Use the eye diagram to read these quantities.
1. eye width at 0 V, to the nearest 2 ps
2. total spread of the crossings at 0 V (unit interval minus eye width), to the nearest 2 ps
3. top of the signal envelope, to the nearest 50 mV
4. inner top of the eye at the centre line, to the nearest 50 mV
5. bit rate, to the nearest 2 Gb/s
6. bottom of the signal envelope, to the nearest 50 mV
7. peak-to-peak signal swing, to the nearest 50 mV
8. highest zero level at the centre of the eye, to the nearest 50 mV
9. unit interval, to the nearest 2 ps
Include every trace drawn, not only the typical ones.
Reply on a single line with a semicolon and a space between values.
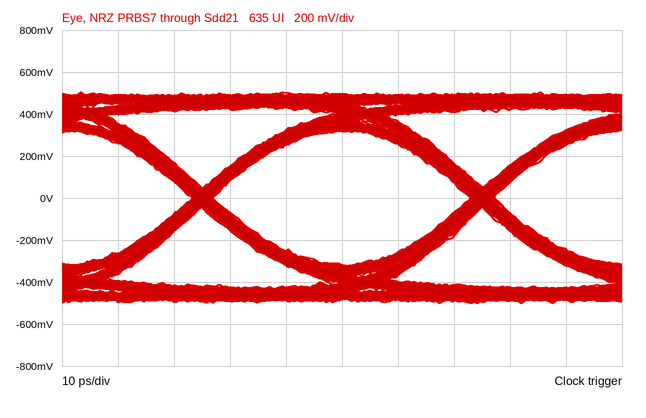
46 ps; 4 ps; 500 mV; 300 mV; 20 Gb/s; -500 mV; 1.00 V; -300 mV; 50 ps
